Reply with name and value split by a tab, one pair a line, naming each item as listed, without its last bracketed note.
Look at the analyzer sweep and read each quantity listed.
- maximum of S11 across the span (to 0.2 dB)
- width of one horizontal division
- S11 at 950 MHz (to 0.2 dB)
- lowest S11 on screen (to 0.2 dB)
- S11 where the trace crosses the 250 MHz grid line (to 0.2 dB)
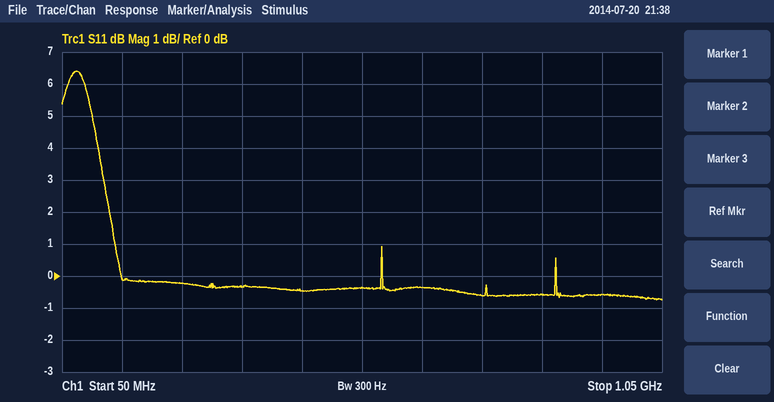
maximum of S11 across the span	6.4 dB
width of one horizontal division	100 MHz
S11 at 950 MHz	-0.6 dB
lowest S11 on screen	-0.8 dB
S11 where the trace crosses the 250 MHz grid line	-0.2 dB
